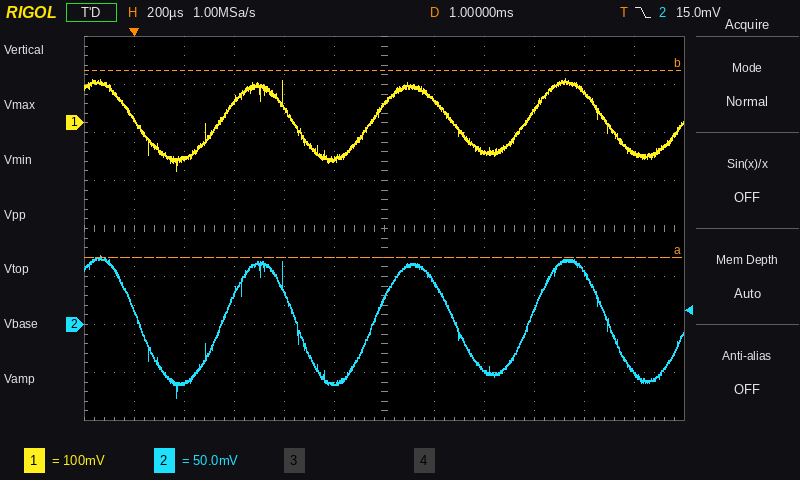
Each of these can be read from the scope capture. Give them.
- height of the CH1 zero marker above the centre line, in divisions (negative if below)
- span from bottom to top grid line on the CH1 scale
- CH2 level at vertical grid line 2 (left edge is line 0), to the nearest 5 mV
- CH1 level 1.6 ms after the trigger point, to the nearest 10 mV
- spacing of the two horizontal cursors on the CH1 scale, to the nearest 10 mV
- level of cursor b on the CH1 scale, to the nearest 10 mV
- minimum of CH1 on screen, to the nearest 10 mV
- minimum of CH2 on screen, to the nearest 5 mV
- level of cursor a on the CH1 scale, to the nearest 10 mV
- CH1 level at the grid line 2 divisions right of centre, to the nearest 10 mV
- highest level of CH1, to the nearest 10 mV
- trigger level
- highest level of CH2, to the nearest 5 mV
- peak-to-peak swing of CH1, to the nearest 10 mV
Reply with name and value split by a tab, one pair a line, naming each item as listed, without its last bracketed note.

height of the CH1 zero marker above the centre line, in divisions	+2.2 div
span from bottom to top grid line on the CH1 scale	800 mV
CH2 level at vertical grid line 2 (left edge is line 0), to the nearest 5 mV	-60 mV
CH1 level 1.6 ms after the trigger point, to the nearest 10 mV	30 mV
spacing of the two horizontal cursors on the CH1 scale, to the nearest 10 mV	390 mV
level of cursor b on the CH1 scale, to the nearest 10 mV	110 mV
minimum of CH1 on screen, to the nearest 10 mV	-100 mV
minimum of CH2 on screen, to the nearest 5 mV	-75 mV
level of cursor a on the CH1 scale, to the nearest 10 mV	-280 mV
CH1 level at the grid line 2 divisions right of centre, to the nearest 10 mV	-60 mV
highest level of CH1, to the nearest 10 mV	90 mV
trigger level	15.0 mV
highest level of CH2, to the nearest 5 mV	70 mV
peak-to-peak swing of CH1, to the nearest 10 mV	190 mV
